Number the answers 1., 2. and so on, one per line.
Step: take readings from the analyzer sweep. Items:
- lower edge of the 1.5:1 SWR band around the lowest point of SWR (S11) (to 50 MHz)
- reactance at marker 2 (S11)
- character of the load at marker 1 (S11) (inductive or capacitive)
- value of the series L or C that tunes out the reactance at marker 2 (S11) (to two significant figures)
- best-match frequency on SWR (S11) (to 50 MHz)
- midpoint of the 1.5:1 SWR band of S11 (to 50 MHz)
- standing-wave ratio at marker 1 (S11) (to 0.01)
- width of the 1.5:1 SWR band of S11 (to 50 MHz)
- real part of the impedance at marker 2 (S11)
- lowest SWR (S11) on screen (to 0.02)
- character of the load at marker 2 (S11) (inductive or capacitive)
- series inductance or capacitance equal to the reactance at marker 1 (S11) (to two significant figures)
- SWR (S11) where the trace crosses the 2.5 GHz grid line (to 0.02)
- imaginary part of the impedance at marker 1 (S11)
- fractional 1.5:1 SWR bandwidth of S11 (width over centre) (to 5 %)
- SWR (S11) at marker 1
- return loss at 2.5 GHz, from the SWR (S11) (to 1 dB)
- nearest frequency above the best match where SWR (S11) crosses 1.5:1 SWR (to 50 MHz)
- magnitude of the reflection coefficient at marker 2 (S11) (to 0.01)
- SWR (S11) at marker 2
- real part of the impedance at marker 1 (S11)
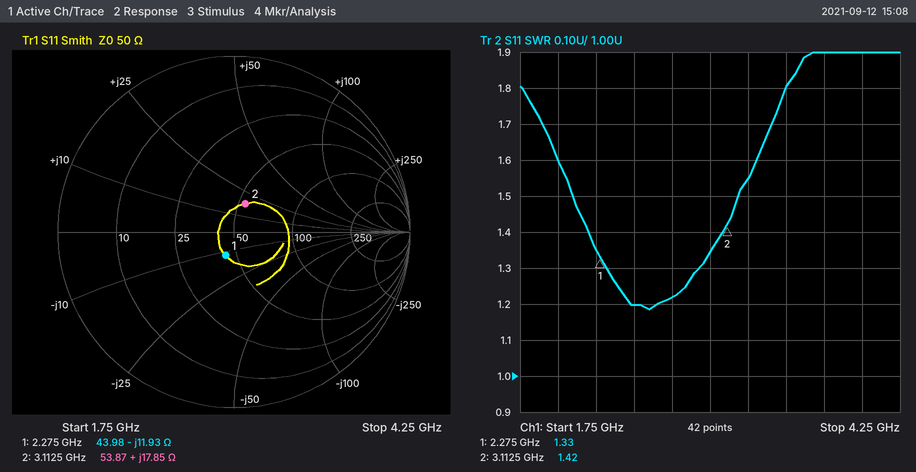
1. 2.10 GHz
2. +17.85 Ω
3. capacitive
4. 2.9 pF
5. 2.60 GHz
6. 2.65 GHz
7. 1.33
8. 1.10 GHz
9. 53.87 Ω
10. 1.18
11. inductive
12. 5.9 pF
13. 1.20
14. -11.93 Ω
15. 40 %
16. 1.33
17. 21 dB
18. 3.20 GHz
19. 0.17
20. 1.42
21. 43.98 Ω
